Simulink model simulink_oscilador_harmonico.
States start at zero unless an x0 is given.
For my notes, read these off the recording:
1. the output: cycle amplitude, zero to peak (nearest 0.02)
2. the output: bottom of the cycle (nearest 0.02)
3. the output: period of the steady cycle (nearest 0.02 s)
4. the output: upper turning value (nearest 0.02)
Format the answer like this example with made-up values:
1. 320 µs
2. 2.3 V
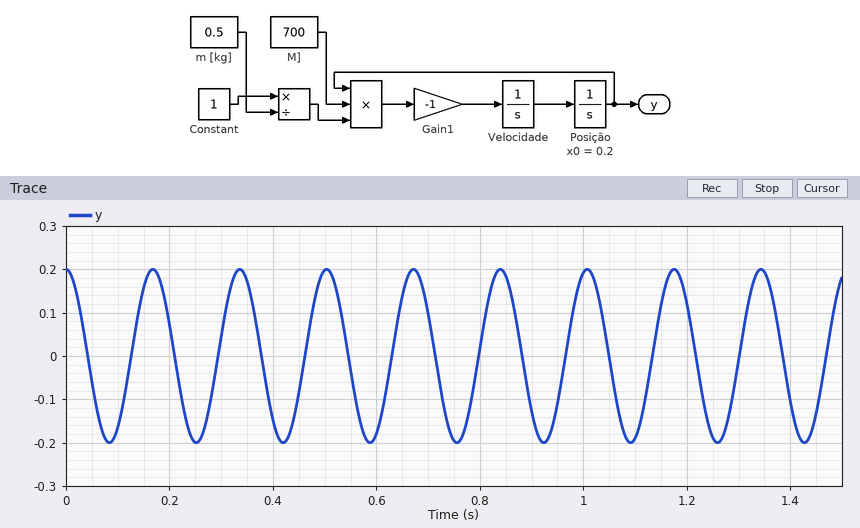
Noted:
1. 0.20
2. -0.20
3. 0.16 s
4. 0.20
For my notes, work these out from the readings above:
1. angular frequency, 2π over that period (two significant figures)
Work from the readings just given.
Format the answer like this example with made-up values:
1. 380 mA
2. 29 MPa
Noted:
1. 39 rad/s
